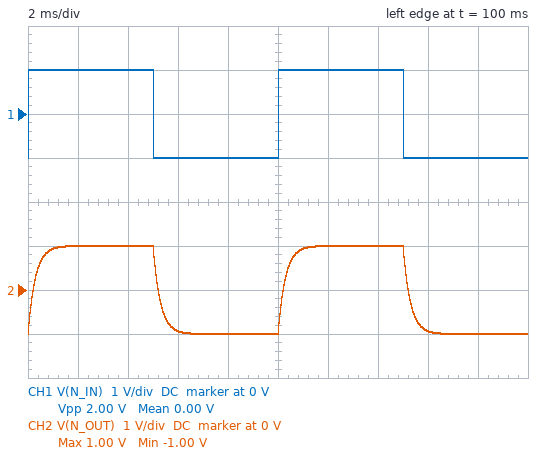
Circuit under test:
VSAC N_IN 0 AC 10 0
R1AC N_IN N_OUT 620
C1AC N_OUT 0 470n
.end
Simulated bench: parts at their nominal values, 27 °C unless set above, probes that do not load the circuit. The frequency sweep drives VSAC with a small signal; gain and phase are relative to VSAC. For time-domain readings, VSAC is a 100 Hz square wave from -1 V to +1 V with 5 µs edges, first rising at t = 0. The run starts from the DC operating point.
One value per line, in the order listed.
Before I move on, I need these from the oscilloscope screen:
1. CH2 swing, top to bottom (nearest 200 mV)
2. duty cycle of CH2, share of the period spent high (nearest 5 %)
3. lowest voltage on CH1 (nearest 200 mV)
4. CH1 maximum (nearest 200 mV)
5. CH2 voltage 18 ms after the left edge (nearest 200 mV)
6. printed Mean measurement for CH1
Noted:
2.0 V
50 %
-1.0 V
1.0 V
-1.0 V
0.00 V
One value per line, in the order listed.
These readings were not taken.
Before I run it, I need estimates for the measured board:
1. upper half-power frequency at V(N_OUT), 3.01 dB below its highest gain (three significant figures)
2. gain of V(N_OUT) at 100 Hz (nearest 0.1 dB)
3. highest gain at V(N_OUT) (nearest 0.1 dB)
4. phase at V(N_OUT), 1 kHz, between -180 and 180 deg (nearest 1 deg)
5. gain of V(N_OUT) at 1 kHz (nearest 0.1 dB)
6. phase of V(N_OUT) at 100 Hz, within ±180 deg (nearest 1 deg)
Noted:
546 Hz
-0.1 dB
0 dB
-61 deg
-6.4 dB
-10 deg
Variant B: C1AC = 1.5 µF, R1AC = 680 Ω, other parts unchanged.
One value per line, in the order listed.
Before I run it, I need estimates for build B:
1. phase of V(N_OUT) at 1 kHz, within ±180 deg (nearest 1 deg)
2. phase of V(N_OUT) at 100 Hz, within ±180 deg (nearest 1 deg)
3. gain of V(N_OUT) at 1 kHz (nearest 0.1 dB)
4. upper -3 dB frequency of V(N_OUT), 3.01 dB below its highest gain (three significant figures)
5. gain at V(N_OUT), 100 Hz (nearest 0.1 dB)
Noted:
-81 deg
-33 deg
-16.2 dB
156 Hz
-1.5 dB
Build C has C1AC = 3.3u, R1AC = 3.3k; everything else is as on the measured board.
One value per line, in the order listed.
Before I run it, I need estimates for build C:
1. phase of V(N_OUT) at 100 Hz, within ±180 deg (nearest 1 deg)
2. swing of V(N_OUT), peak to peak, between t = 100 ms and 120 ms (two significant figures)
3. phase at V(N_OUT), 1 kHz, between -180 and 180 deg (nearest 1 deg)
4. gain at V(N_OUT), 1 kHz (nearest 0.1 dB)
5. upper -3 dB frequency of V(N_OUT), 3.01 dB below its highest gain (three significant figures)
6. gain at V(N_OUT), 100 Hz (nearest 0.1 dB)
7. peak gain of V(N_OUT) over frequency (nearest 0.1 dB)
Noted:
-82 deg
450 mV
-89 deg
-36.7 dB
14.6 Hz
-16.8 dB
0 dB
